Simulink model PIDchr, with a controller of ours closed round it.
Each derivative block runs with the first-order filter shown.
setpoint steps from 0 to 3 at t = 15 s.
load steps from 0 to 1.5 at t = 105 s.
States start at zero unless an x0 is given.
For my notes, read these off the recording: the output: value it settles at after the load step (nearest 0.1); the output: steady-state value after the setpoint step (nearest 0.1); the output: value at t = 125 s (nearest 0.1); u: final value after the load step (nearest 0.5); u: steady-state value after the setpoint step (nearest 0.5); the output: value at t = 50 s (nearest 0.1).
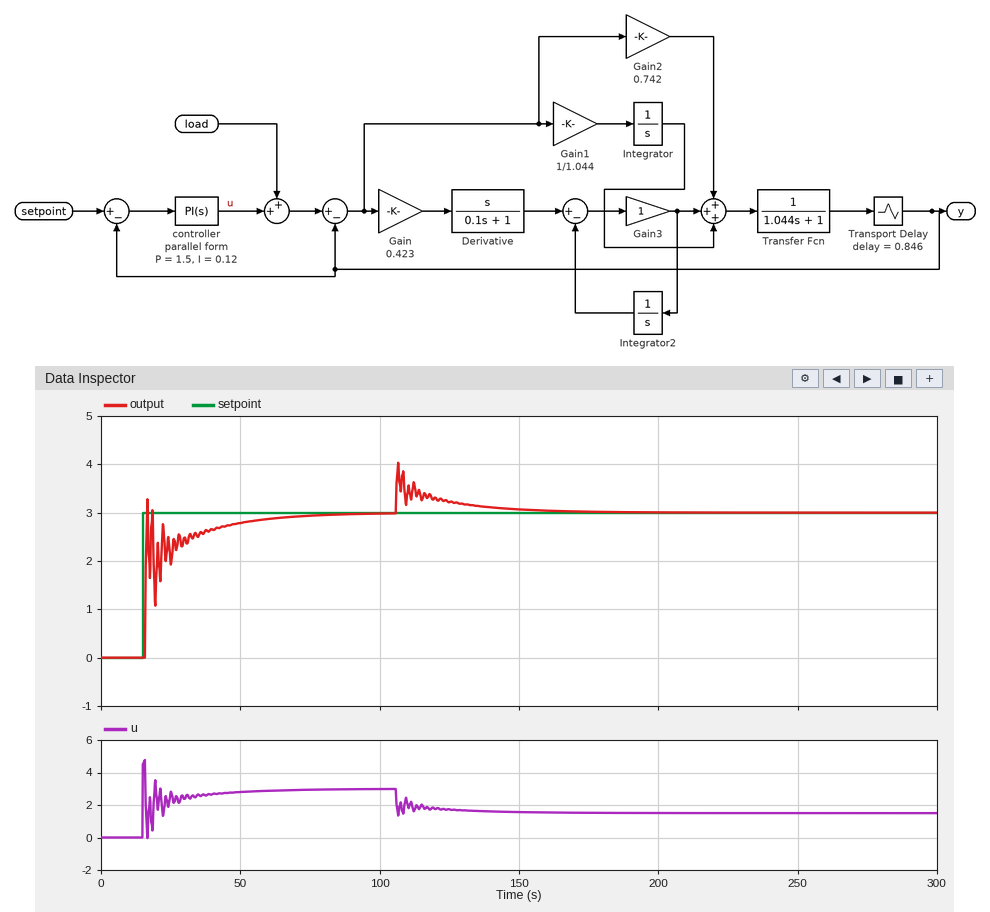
3.0
3.0
3.2
1.5
3.0
2.8
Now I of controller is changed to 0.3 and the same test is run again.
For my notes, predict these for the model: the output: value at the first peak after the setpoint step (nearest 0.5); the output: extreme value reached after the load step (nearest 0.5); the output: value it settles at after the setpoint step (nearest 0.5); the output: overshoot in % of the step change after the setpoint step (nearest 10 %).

3.5
4.0
3.0
20 %
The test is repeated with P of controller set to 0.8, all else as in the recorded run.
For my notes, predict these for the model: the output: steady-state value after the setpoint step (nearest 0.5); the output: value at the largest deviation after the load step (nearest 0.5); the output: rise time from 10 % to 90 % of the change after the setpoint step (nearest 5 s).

3.0
4.0
25 s
